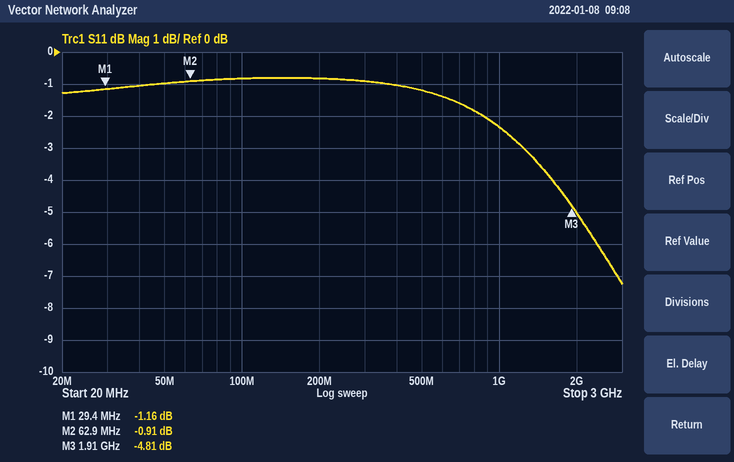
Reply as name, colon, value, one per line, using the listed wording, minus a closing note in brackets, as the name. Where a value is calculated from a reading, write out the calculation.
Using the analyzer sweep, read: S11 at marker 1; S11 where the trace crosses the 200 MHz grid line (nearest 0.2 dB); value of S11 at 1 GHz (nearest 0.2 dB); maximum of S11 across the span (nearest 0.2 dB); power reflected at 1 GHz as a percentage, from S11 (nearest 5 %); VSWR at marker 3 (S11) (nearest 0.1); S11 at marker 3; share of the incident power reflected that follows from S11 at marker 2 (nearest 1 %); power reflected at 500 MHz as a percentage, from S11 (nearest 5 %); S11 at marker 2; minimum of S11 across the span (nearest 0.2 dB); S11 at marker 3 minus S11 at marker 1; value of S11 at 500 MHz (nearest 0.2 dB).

S11 at marker 1: -1.16 dB
S11 where the trace crosses the 200 MHz grid line: -0.8 dB
value of S11 at 1 GHz: -2.4 dB
maximum of S11 across the span: -0.8 dB
power reflected at 1 GHz as a percentage, from S11: 10^(-2.4/10) ≈ 57.5 %, so 60 % to the nearest 5 %
VSWR at marker 3 (S11): (1 + 0.5748)/(1 − 0.5748) ≈ 3.7
S11 at marker 3: -4.81 dB
share of the incident power reflected that follows from S11 at marker 2: 10^(-0.91/10) ≈ 81 %
power reflected at 500 MHz as a percentage, from S11: 10^(-1.2/10) ≈ 75.9 %, so 75 % to the nearest 5 %
S11 at marker 2: -0.91 dB
minimum of S11 across the span: -7.2 dB
S11 at marker 3 minus S11 at marker 1: -4.81 − (-1.16) = -3.65 dB
value of S11 at 500 MHz: -1.2 dB
